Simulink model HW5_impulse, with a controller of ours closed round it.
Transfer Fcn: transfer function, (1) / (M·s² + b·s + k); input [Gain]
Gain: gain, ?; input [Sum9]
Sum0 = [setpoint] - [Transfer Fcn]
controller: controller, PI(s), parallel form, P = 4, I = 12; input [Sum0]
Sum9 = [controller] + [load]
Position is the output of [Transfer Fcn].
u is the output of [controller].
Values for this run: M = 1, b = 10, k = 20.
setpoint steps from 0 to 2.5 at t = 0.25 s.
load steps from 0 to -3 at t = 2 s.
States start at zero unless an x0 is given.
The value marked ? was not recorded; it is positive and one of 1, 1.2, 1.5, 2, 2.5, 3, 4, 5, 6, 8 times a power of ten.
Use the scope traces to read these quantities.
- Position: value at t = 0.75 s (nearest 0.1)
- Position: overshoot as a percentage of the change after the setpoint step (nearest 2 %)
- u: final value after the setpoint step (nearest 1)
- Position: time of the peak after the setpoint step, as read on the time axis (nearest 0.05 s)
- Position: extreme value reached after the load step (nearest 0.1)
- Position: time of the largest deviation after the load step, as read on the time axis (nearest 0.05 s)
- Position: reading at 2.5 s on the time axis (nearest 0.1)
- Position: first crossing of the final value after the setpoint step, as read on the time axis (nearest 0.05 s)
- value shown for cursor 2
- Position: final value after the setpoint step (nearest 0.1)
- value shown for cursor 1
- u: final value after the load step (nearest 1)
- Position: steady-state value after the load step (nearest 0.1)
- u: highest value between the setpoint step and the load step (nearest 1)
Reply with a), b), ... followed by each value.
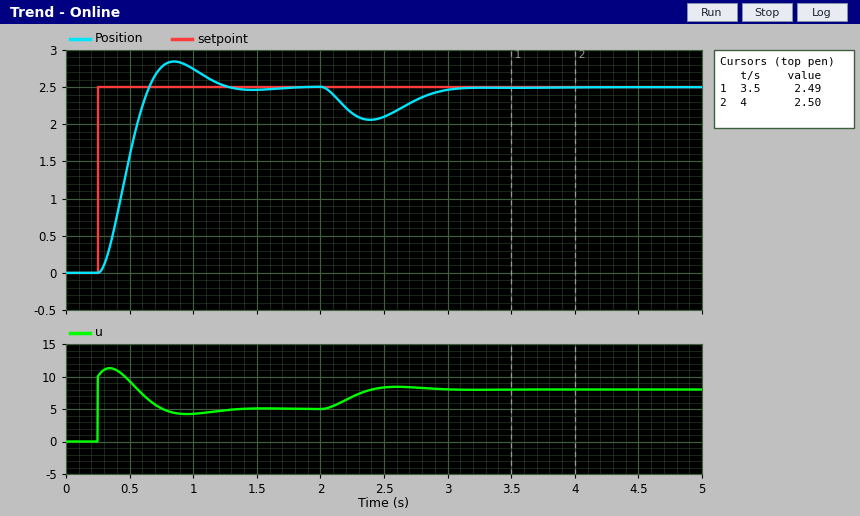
a) 2.8
b) 14 %
c) 5
d) 0.85 s
e) 2.1
f) 2.40 s
g) 2.1
h) 0.65 s
i) 2.50
j) 2.5
k) 2.49
l) 8
m) 2.5
n) 11
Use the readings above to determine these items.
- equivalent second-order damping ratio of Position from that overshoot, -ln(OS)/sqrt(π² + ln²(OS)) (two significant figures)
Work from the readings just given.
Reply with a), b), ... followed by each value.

a) 0.53
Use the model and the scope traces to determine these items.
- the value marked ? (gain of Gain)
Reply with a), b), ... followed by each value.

a) 10
